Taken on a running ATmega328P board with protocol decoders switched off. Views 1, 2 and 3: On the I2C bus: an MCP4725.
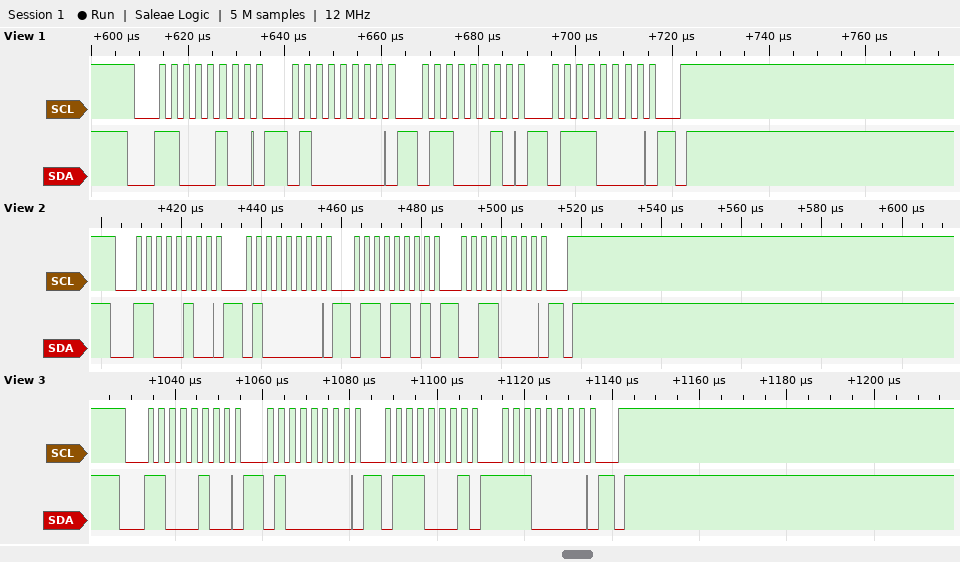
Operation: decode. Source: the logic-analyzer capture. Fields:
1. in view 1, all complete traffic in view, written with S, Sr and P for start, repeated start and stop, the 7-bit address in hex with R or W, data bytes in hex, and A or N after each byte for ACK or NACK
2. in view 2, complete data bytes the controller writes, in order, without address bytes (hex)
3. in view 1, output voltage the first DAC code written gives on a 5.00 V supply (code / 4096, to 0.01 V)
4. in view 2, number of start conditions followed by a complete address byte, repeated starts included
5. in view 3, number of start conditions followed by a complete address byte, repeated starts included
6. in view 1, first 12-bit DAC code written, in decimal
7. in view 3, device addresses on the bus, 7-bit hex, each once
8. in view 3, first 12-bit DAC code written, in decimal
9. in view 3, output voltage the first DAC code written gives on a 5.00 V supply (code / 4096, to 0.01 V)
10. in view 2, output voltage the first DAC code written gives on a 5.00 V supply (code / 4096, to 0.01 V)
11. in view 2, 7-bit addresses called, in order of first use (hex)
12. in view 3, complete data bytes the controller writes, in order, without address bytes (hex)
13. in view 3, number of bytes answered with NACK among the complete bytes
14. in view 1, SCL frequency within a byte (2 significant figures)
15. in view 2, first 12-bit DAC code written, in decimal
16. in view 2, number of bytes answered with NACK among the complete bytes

S 62W A 40 A 62 A 70 A P
40 6D 30
1.92 V
1
1
1575
0x62
1822
2.22 V
2.13 V
0x62
40 71 E0
0
400 kHz
1747
0
